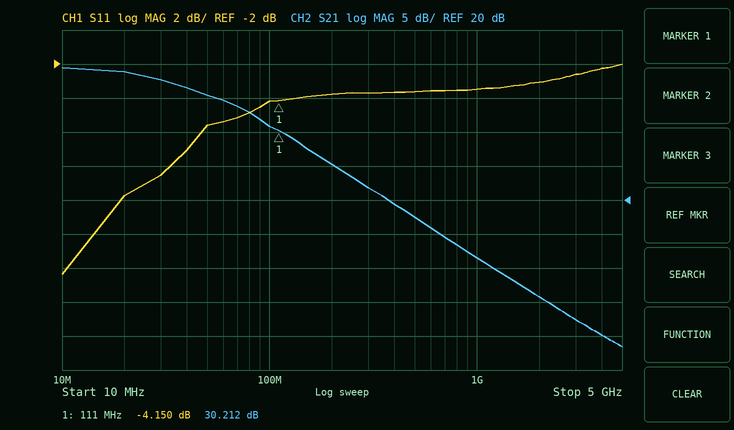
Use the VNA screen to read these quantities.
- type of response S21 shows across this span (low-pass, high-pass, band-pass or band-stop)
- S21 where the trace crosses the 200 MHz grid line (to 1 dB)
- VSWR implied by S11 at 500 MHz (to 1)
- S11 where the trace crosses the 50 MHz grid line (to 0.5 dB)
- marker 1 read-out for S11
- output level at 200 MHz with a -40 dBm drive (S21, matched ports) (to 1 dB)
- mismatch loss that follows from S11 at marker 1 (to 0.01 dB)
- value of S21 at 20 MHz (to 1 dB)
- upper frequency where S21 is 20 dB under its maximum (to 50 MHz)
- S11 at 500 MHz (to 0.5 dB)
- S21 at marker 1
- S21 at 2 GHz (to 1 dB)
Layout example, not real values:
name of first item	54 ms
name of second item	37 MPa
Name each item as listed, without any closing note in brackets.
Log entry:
type of response S21 shows across this span	low-pass
S21 where the trace crosses the 200 MHz grid line	25 dB
VSWR implied by S11 at 500 MHz	5
S11 where the trace crosses the 50 MHz grid line	-5.5 dB
marker 1 read-out for S11	-4.150 dB
output level at 200 MHz with a -40 dBm drive (S21, matched ports)	-15 dBm
mismatch loss that follows from S11 at marker 1	2.11 dB
value of S21 at 20 MHz	39 dB
upper frequency where S21 is 20 dB under its maximum	400 MHz
S11 at 500 MHz	-3.5 dB
S21 at marker 1	30.212 dB
S21 at 2 GHz	6 dB
